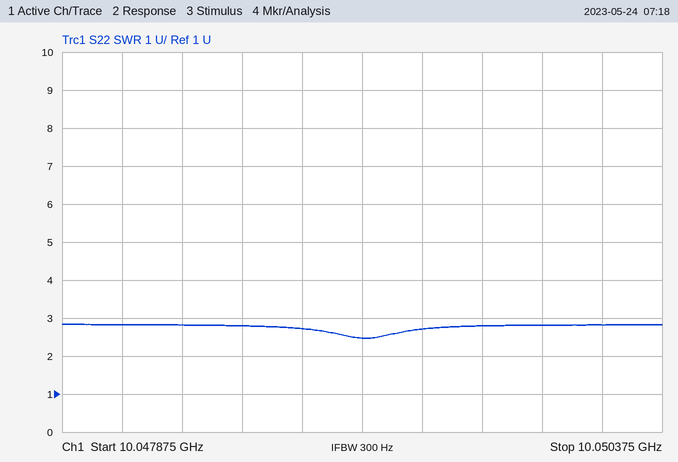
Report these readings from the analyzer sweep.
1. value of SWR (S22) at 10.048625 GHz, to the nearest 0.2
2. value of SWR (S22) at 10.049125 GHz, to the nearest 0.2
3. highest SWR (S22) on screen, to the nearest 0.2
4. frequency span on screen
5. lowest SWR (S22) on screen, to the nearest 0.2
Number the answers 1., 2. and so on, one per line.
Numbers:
1. 2.8
2. 2.4
3. 2.8
4. 2.5 MHz
5. 2.4
